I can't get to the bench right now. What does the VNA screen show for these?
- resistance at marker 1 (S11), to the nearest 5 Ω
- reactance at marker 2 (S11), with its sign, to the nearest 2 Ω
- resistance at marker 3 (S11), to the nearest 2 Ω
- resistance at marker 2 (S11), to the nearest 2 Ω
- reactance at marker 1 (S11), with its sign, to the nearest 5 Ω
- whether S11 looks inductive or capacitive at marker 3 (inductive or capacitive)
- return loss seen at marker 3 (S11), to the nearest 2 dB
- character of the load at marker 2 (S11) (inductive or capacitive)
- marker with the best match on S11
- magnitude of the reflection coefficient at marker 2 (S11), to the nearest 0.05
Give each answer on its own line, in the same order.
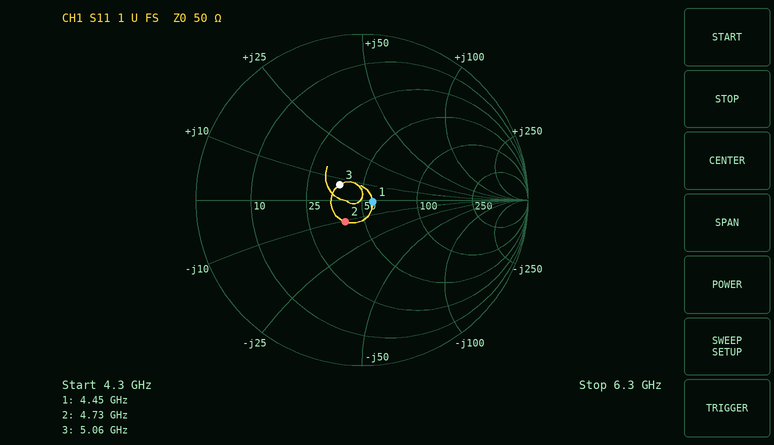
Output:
55 Ω
-10 Ω
38 Ω
40 Ω
0 Ω
inductive
16 dB
capacitive
marker 1
0.15
